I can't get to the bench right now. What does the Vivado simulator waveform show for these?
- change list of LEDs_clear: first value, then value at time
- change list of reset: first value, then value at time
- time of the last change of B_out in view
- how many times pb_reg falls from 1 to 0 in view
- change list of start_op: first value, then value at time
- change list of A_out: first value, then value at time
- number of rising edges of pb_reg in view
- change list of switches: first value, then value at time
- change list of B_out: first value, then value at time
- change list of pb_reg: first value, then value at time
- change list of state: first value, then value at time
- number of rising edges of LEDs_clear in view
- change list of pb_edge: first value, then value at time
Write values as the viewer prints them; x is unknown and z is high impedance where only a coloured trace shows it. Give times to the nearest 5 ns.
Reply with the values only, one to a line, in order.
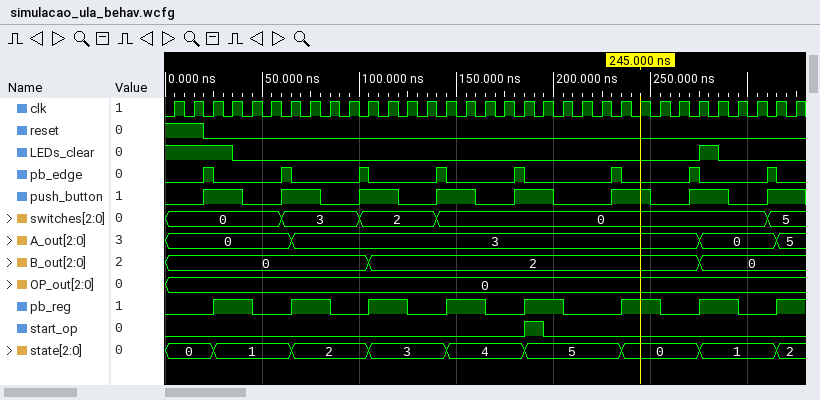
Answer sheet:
1, 0 at 35 ns, 1 at 275 ns, 0 at 285 ns
1, 0 at 20 ns
275 ns
7
0, 1 at 185 ns, 0 at 195 ns
0, 3 at 65 ns, 0 at 275 ns, 5 at 315 ns
8
0, 3 at 60 ns, 2 at 100 ns, 0 at 140 ns, 5 at 310 ns
0, 2 at 105 ns, 0 at 275 ns
0, 1 at 25 ns, 0 at 45 ns, 1 at 65 ns, 0 at 85 ns, 1 at 105 ns, 0 at 125 ns, 1 at 145 ns, 0 at 165 ns, 1 at 185 ns, 0 at 205 ns, 1 at 235 ns, 0 at 255 ns, 1 at 275 ns, 0 at 295 ns, 1 at 315 ns
0, 1 at 25 ns, 2 at 65 ns, 3 at 105 ns, 4 at 145 ns, 5 at 185 ns, 0 at 235 ns, 1 at 275 ns, 2 at 315 ns
1
0, 1 at 20 ns, 0 at 25 ns, 1 at 60 ns, 0 at 65 ns, 1 at 100 ns, 0 at 105 ns, 1 at 140 ns, 0 at 145 ns, 1 at 180 ns, 0 at 185 ns, 1 at 230 ns, 0 at 235 ns, 1 at 270 ns, 0 at 275 ns, 1 at 310 ns, 0 at 315 ns
